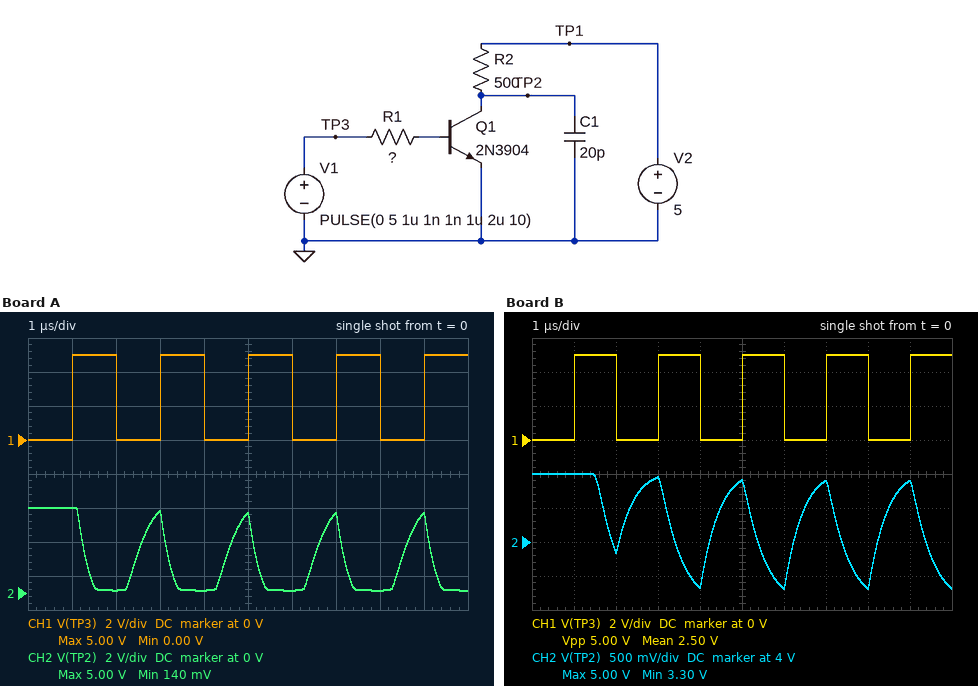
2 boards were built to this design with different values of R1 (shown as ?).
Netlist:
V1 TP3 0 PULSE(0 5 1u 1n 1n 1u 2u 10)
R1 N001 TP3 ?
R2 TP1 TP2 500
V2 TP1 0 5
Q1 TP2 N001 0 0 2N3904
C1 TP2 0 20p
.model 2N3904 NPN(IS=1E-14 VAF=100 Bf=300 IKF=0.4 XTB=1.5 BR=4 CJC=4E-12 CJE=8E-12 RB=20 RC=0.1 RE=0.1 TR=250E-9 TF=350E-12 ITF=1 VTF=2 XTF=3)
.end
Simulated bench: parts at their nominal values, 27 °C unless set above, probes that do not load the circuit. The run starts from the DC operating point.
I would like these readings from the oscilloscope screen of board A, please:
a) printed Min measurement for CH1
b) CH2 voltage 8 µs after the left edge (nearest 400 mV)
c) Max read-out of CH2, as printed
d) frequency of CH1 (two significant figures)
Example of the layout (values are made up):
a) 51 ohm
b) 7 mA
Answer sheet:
a) 0.00 V
b) 0 V
c) 5.00 V
d) 500 kHz
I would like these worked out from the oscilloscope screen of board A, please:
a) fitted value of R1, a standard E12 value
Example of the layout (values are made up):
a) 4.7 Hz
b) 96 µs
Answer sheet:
a) 68 kΩ
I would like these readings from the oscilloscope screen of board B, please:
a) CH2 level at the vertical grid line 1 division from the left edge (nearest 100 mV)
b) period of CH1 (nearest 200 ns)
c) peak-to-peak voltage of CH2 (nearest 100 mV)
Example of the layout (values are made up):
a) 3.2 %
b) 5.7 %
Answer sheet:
a) 5.0 V
b) 2.0 µs
c) 1.7 V
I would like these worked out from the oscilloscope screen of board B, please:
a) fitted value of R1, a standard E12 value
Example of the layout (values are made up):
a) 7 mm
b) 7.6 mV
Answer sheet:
a) 330 kΩ
